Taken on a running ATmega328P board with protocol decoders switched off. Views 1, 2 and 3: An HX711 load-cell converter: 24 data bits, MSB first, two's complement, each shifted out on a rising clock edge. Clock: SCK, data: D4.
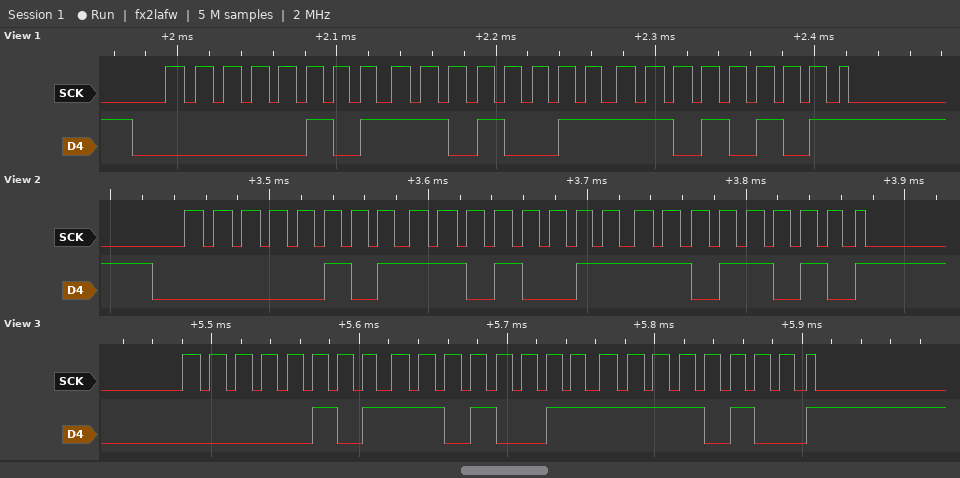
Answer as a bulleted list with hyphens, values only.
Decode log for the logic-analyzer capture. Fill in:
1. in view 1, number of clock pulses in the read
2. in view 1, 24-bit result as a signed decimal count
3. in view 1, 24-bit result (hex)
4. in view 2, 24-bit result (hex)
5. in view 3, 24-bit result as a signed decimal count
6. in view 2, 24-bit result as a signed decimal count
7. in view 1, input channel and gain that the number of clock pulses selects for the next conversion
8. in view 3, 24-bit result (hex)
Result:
- 25
- 381909
- 0x05D3D5
- 0x05D3DA
- 381940
- 381914
- channel A, gain 128
- 0x05D3F4
